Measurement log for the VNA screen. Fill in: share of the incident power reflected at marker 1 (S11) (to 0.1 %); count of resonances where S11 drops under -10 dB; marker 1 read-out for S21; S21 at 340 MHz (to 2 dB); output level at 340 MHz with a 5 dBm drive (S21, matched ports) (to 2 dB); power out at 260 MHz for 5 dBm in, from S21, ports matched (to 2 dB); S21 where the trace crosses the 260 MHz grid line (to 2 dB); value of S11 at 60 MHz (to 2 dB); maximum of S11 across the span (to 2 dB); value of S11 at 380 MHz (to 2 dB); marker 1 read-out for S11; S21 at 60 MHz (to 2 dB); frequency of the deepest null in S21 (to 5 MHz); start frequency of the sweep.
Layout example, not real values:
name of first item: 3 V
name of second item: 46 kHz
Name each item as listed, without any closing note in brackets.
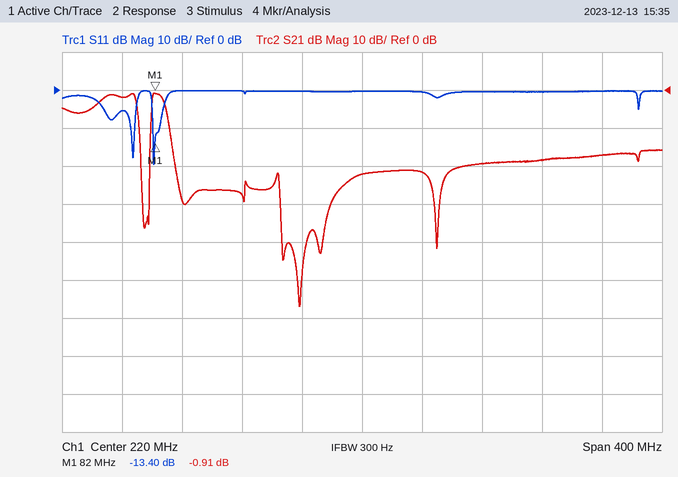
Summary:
share of the incident power reflected at marker 1 (S11): 4.6 %
count of resonances where S11 drops under -10 dB: 2
marker 1 read-out for S21: -0.91 dB
S21 at 340 MHz: -18 dB
output level at 340 MHz with a 5 dBm drive (S21, matched ports): -14 dBm
power out at 260 MHz for 5 dBm in, from S21, ports matched: -16 dBm
S21 where the trace crosses the 260 MHz grid line: -22 dB
value of S11 at 60 MHz: -6 dB
maximum of S11 across the span: 0 dB
value of S11 at 380 MHz: 0 dB
marker 1 read-out for S11: -13.40 dB
S21 at 60 MHz: -2 dB
frequency of the deepest null in S21: 180 MHz
start frequency of the sweep: 20 MHz
